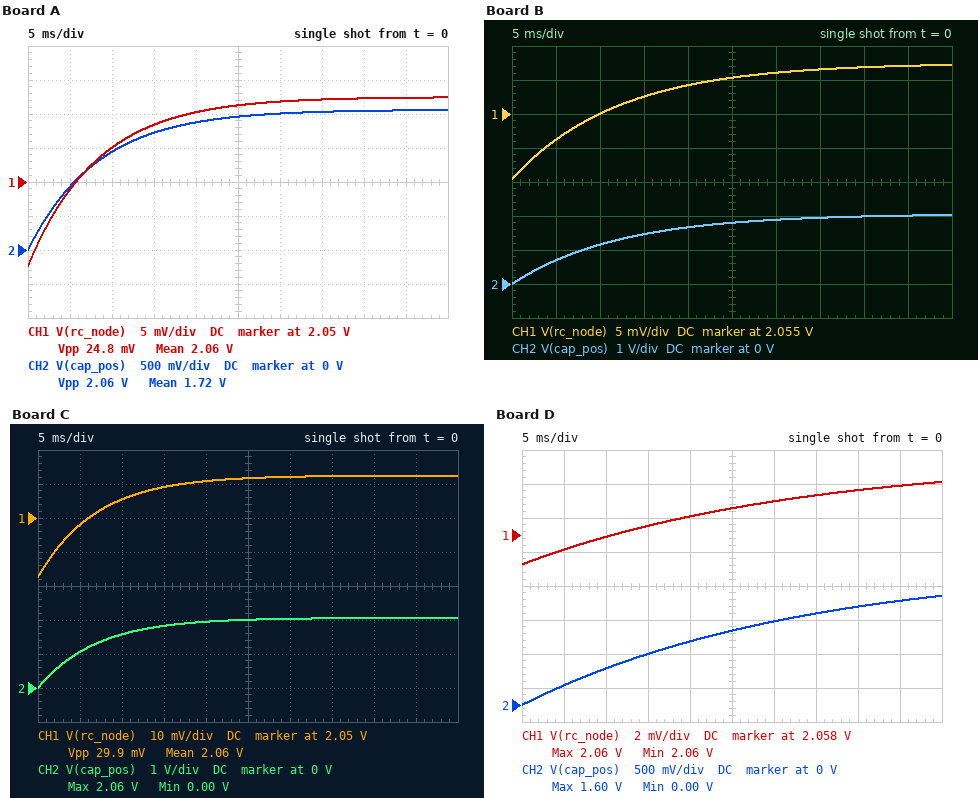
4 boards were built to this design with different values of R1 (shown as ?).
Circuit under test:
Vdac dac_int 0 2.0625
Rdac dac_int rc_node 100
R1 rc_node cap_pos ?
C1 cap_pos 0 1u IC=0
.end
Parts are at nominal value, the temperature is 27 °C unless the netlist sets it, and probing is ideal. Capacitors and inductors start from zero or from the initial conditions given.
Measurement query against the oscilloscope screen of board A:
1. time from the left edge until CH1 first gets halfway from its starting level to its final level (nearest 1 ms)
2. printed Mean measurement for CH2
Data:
6 ms
1.72 V
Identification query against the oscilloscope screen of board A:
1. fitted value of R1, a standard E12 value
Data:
8.2 kΩ
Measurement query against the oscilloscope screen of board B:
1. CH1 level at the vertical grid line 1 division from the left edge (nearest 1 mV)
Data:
2.051 V
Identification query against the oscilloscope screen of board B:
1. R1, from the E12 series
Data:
12 kΩ
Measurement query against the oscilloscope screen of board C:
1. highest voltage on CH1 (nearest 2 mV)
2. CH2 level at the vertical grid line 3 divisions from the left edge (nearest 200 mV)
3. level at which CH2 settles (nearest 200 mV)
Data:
2.062 V
1.8 V
2.0 V
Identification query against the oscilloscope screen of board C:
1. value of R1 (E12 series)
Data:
6.8 kΩ
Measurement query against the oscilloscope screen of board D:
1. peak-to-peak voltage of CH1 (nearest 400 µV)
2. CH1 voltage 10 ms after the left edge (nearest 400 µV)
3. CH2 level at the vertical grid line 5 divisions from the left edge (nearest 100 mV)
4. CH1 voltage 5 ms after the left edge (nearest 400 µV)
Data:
4.8 mV
2.0580 V
1.1 V
2.0572 V
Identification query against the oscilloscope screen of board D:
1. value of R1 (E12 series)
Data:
33 kΩ
